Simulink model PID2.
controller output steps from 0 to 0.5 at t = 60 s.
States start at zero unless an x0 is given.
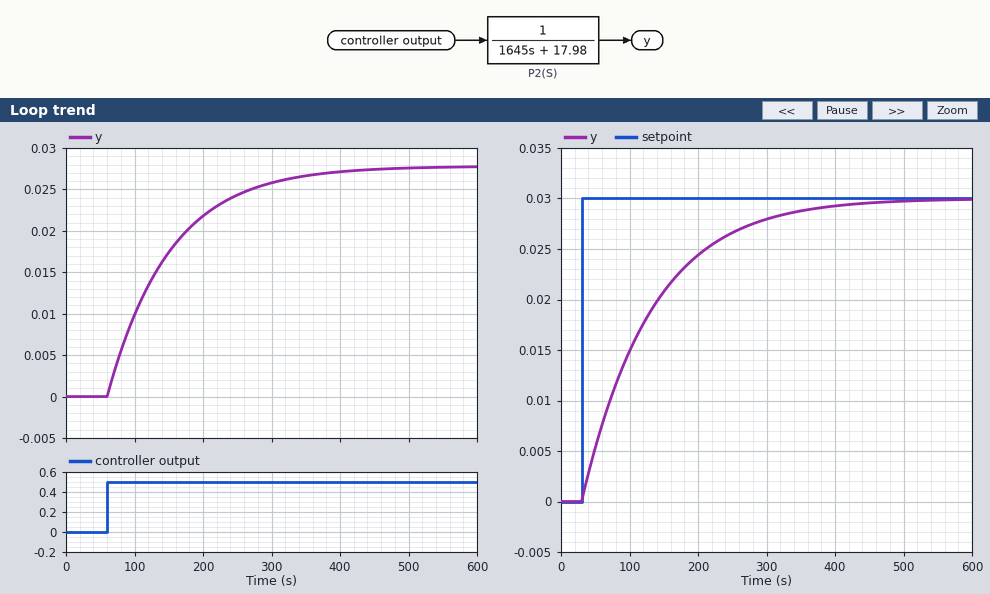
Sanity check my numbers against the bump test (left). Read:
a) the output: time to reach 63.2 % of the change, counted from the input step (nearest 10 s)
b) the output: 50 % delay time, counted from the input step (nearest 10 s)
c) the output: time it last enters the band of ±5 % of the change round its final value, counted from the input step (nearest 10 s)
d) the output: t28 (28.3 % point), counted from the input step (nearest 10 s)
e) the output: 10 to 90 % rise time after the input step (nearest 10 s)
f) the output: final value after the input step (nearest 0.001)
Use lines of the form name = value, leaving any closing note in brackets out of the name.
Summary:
the output: time to reach 63.2 % of the change, counted from the input step = 90 s
the output: 50 % delay time, counted from the input step = 60 s
the output: time it last enters the band of ±5 % of the change round its final value, counted from the input step = 270 s
the output: t28 (28.3 % point), counted from the input step = 30 s
the output: 10 to 90 % rise time after the input step = 200 s
the output: final value after the input step = 0.028
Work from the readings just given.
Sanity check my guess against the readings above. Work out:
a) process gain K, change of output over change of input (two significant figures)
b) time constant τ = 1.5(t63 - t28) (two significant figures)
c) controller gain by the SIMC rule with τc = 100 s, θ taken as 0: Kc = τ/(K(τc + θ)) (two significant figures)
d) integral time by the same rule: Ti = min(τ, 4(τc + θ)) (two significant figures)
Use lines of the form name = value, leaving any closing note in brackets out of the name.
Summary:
process gain K, change of output over change of input = 0.056
time constant τ = 1.5(t63 - t28) = 90 s
controller gain by the SIMC rule with τc = 100 s, θ taken as 0: Kc = τ/(K(τc + θ)) = 16
integral time by the same rule: Ti = min(τ, 4(τc + θ)) = 90 s
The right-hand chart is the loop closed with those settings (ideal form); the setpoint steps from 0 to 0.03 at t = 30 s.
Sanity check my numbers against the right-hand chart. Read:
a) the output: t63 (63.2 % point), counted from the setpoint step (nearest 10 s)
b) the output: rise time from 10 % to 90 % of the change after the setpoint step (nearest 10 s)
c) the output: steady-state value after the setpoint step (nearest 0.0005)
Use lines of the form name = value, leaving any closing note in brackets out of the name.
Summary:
the output: t63 (63.2 % point), counted from the setpoint step = 100 s
the output: rise time from 10 % to 90 % of the change after the setpoint step = 220 s
the output: steady-state value after the setpoint step = 0.0300
